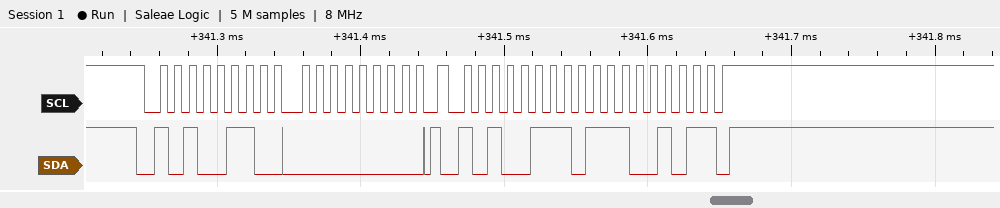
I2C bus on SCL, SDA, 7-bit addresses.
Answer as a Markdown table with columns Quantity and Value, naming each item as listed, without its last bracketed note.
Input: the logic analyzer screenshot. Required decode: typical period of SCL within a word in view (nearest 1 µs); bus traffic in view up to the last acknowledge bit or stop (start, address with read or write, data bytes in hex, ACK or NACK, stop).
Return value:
| Quantity | Value |
|---|---|
| typical period of SCL within a word in view | 10 µs |
| bus traffic in view up to the last acknowledge bit or stop | start, address 53 write ACK, 00 ACK, repeated start, address 53 read ACK, E5 NACK, stop |
